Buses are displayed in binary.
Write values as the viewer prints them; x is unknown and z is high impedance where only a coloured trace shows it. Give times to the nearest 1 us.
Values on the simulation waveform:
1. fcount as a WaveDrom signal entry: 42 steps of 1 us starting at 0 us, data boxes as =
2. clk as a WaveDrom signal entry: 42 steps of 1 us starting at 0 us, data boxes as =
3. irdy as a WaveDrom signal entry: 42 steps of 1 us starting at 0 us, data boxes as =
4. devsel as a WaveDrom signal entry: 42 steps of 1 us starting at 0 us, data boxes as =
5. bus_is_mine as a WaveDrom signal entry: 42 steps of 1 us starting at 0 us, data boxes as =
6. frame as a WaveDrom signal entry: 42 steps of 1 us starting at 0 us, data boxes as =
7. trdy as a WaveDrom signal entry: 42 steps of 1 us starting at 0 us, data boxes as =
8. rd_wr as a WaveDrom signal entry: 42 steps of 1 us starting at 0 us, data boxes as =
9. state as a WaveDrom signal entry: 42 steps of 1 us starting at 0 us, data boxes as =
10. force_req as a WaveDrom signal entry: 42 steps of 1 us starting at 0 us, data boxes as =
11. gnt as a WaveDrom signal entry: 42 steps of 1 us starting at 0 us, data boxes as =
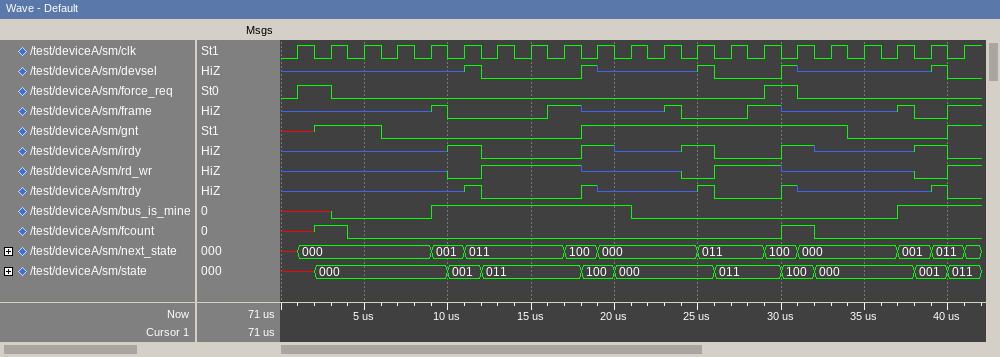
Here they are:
{name: 'fcount', wave: 'x.1.0.........................1.0.........'}
{name: 'clk', wave: '010101010101010101010101010101010101010101'}
{name: 'irdy', wave: 'z.........1.0.....1.z...1.0...1.z.....1.0.'}
{name: 'devsel', wave: 'z..........10.....1z.....10...1z.......10.'}
{name: 'bus_is_mine', wave: 'x..0.....1...........0...............1....'}
{name: 'frame', wave: 'z........10.....1.z....10...1.z......10.1.'}
{name: 'trdy', wave: 'z..........10.....1z.....10...1z.......10.'}
{name: 'rd_wr', wave: 'z.........0.1.....z.....0.1...z.......0.1.'}
{name: 'state', wave: 'x.=.......=.=.....=.=.....=...=.=.....=.=.', data: '000 001 011 100 000 011 100 000 001 011'}
{name: 'force_req', wave: '01.0.........................1.0..........'}
{name: 'gnt', wave: 'x.1...0...........1...............0.....1.'}
